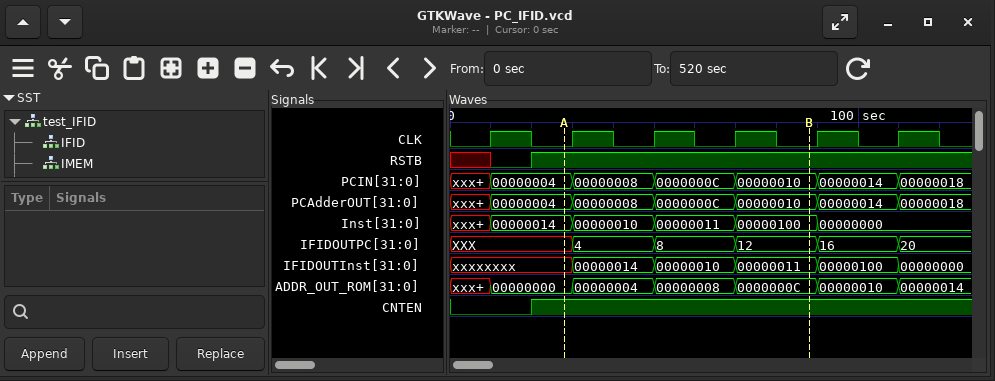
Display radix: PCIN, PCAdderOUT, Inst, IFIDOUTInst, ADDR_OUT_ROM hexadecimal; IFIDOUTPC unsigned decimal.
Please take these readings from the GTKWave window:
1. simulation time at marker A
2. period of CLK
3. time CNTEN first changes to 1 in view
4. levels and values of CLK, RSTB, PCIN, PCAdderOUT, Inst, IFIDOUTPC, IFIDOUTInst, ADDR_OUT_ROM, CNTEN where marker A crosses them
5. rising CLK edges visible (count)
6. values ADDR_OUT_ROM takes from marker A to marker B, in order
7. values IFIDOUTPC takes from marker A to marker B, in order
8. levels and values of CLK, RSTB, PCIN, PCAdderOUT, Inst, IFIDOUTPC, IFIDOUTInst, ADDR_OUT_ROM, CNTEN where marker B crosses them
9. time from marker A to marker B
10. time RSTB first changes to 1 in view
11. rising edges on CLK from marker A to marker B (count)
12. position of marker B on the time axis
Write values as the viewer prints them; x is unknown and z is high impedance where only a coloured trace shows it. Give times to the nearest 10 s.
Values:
30 s
20 s
20 s
CLK=0, RSTB=1, PCIN=00000004, PCAdderOUT=00000004, Inst=00000014, IFIDOUTPC=XXX, IFIDOUTInst=xxxxxxxx, ADDR_OUT_ROM=00000000, CNTEN=1
6
00000000, 00000004, 00000008, 0000000C
XXX, 4, 8, 12
CLK=0, RSTB=1, PCIN=00000010, PCAdderOUT=00000010, Inst=00000100, IFIDOUTPC=12, IFIDOUTInst=00000011, ADDR_OUT_ROM=0000000C, CNTEN=1
60 s
20 s
3
90 s
